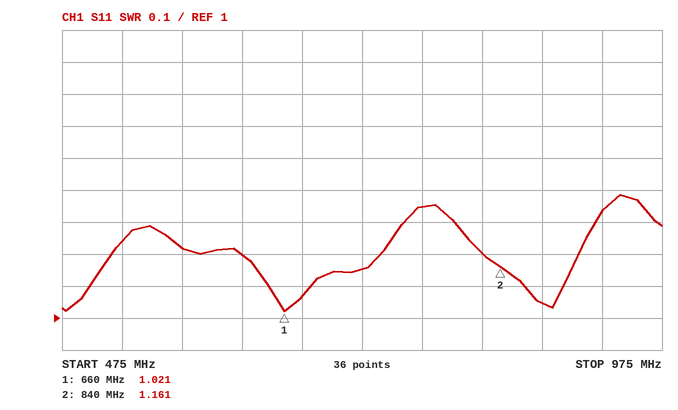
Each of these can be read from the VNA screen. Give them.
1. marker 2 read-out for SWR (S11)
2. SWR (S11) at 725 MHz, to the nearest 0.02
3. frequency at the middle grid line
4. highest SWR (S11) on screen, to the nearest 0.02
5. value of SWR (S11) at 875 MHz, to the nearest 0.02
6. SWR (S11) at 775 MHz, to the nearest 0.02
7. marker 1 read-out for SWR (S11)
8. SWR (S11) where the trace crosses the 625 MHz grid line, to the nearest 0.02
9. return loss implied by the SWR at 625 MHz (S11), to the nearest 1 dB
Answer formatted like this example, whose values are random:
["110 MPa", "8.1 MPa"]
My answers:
["1.161", "1.16", "725 MHz", "1.38", "1.04", "1.34", "1.021", "1.20", "21 dB"]
